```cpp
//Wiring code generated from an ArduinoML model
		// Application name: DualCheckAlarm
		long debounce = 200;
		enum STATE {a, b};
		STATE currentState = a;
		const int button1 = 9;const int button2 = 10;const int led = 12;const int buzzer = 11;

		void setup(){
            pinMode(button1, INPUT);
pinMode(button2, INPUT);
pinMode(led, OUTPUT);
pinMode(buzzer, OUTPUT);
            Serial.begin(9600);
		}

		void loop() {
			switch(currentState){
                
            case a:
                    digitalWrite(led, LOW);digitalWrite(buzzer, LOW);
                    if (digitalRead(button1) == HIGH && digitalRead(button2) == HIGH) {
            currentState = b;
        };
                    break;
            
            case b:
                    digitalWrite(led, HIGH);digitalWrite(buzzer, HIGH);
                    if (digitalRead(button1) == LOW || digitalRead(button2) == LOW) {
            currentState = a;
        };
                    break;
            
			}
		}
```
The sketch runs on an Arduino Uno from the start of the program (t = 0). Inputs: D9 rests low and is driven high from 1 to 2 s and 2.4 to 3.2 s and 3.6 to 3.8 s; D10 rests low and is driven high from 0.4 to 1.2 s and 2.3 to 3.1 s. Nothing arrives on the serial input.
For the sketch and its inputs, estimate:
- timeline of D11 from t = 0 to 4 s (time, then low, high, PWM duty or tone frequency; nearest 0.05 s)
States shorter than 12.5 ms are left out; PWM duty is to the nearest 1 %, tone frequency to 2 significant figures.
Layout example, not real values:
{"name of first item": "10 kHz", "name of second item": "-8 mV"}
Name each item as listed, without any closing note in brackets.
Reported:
{"timeline of D11 from t = 0 to 4 s": "0 s low; 1 s high; 1.2 s low; 2.4 s high; 3.1 s low"}
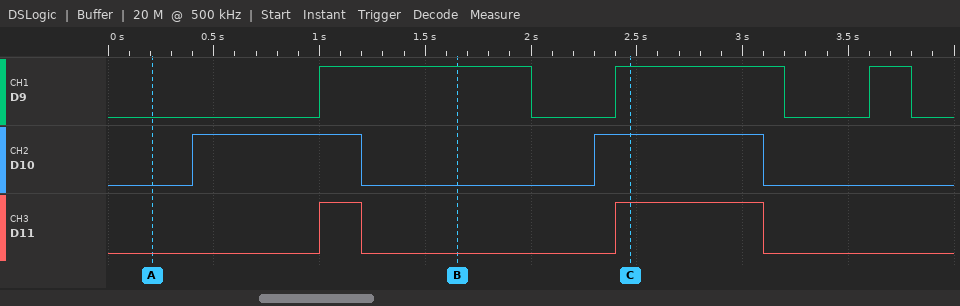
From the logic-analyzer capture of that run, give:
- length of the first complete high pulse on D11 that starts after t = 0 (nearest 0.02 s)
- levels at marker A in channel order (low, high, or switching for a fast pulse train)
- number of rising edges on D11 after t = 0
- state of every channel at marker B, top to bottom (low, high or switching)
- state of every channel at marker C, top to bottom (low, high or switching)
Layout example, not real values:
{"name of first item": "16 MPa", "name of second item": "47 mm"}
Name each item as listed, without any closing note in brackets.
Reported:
{"length of the first complete high pulse on D11 that starts after t = 0": "0.20 s", "levels at marker A in channel order": "D9 low, D10 low, D11 low", "number of rising edges on D11 after t = 0": "2", "state of every channel at marker B, top to bottom": "D9 high, D10 low, D11 low", "state of every channel at marker C, top to bottom": "D9 high, D10 high, D11 high"}
